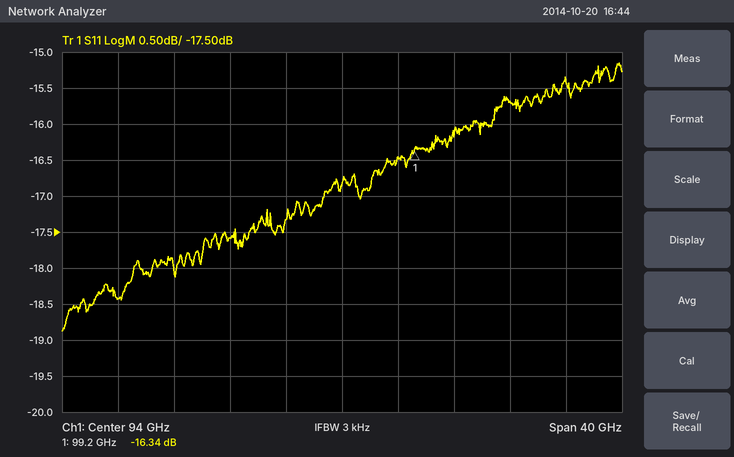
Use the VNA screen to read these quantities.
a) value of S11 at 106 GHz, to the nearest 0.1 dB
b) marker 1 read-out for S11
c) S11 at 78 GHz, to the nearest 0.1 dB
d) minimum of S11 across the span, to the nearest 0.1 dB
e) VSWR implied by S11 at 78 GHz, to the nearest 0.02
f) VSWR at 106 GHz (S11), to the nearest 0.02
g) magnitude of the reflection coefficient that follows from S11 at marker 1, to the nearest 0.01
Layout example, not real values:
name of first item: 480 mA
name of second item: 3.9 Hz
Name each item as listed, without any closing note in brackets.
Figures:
value of S11 at 106 GHz, to the nearest 0.1 dB: -15.7 dB
marker 1 read-out for S11: -16.34 dB
S11 at 78 GHz, to the nearest 0.1 dB: -18.4 dB
minimum of S11 across the span, to the nearest 0.1 dB: -18.9 dB
VSWR implied by S11 at 78 GHz, to the nearest 0.02: 1.28
VSWR at 106 GHz (S11), to the nearest 0.02: 1.40
magnitude of the reflection coefficient that follows from S11 at marker 1, to the nearest 0.01: 0.15
